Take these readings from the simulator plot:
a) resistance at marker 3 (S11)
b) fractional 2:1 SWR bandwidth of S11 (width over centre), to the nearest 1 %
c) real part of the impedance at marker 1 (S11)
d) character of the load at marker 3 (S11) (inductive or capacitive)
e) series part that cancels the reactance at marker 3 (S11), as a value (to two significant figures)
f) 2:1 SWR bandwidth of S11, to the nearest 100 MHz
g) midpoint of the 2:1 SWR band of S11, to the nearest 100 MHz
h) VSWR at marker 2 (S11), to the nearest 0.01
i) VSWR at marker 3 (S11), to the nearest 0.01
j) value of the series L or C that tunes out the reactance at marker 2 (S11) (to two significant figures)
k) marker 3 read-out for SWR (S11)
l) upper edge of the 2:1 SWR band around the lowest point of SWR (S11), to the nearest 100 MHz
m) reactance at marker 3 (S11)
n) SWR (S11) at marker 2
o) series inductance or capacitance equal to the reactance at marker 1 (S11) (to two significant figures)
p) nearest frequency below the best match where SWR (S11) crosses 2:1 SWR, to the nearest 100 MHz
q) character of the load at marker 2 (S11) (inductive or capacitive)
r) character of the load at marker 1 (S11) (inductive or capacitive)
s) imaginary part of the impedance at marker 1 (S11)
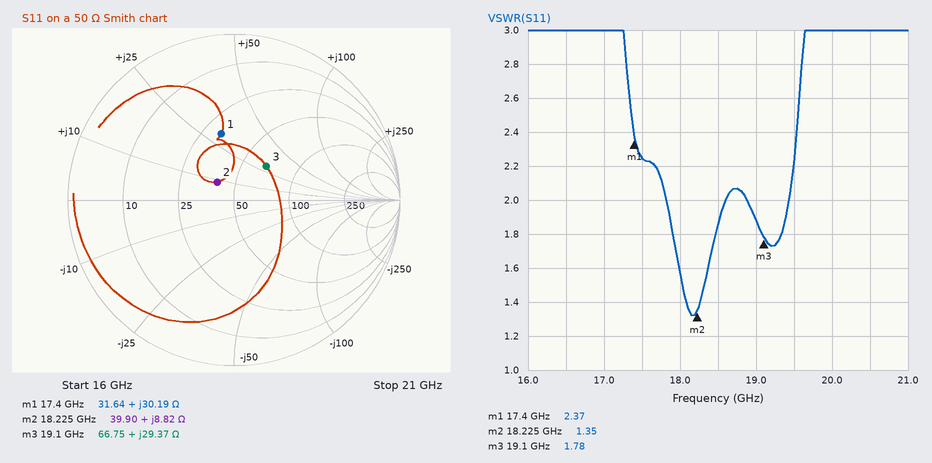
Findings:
66.75 Ω
4 %
31.64 Ω
inductive
280 fF
800 MHz
18.2 GHz
1.35
1.78
990 fF
1.78
18.6 GHz
+29.37 Ω
1.35
280 pH
17.8 GHz
inductive
inductive
+30.19 Ω
